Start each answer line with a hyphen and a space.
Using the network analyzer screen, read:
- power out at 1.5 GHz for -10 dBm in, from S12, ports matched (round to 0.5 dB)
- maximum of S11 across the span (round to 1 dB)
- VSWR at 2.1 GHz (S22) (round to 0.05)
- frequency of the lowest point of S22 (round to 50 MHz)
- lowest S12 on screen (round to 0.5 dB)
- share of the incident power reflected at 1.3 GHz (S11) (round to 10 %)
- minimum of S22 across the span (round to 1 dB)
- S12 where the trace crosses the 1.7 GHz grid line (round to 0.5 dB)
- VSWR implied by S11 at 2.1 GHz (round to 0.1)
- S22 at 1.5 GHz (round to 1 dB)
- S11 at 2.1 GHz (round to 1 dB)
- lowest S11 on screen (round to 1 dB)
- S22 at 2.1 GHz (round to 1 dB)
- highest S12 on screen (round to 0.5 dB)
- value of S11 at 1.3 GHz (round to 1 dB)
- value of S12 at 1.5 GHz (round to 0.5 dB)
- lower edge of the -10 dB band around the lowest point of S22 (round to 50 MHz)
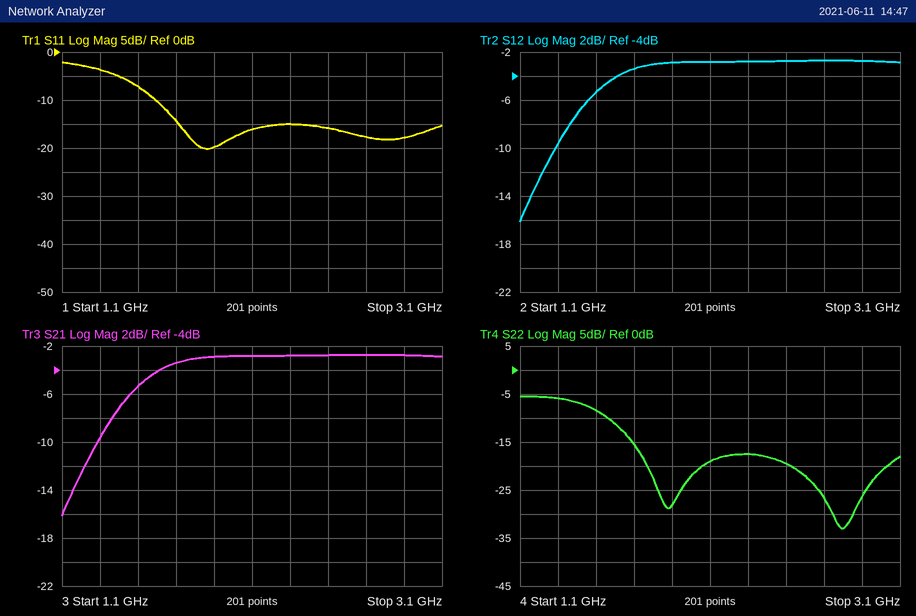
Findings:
- -15.5 dBm
- -2 dB
- 1.25
- 2.80 GHz
- -16.0 dB
- 40 %
- -33 dB
- -3.5 dB
- 1.4
- -8 dB
- -16 dB
- -20 dB
- -19 dB
- -2.5 dB
- -4 dB
- -5.5 dB
- 1.55 GHz
